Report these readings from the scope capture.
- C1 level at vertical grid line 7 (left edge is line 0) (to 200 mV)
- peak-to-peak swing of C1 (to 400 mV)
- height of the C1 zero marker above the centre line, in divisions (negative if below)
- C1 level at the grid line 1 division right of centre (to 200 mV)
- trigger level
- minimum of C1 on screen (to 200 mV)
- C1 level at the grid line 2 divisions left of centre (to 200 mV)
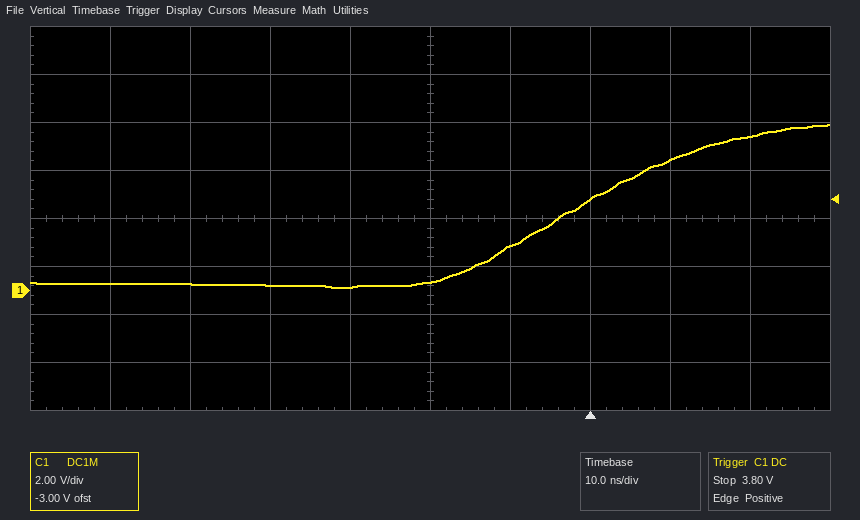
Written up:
3.8 V
6.8 V
-1.5 div
1.8 V
3.80 V
200 mV
200 mV
